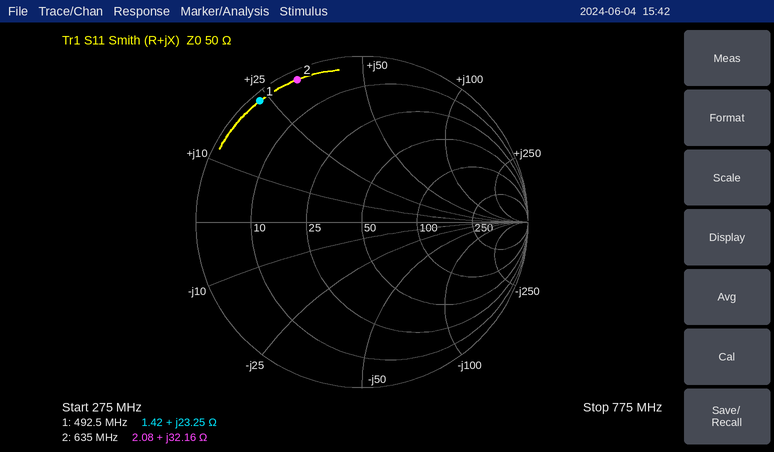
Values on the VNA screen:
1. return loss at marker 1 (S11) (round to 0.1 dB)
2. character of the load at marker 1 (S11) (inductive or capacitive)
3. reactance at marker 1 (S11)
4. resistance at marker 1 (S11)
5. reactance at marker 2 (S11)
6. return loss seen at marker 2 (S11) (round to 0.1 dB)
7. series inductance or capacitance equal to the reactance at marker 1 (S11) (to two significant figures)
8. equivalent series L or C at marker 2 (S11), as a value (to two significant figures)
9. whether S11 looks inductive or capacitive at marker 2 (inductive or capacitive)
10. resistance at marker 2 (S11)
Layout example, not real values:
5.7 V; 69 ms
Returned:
0.4 dB; inductive; +23.25 Ω; 1.42 Ω; +32.16 Ω; 0.5 dB; 7.5 nH; 8.1 nH; inductive; 2.08 Ω
